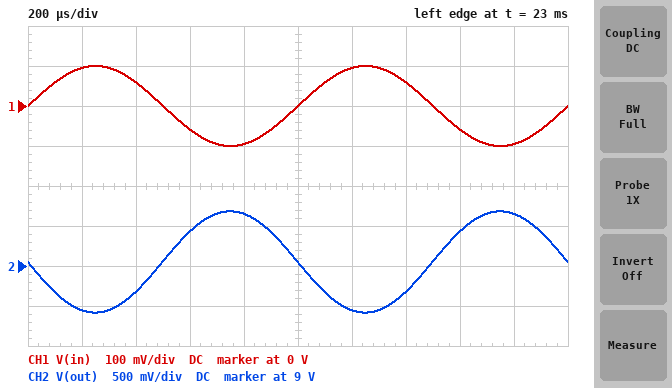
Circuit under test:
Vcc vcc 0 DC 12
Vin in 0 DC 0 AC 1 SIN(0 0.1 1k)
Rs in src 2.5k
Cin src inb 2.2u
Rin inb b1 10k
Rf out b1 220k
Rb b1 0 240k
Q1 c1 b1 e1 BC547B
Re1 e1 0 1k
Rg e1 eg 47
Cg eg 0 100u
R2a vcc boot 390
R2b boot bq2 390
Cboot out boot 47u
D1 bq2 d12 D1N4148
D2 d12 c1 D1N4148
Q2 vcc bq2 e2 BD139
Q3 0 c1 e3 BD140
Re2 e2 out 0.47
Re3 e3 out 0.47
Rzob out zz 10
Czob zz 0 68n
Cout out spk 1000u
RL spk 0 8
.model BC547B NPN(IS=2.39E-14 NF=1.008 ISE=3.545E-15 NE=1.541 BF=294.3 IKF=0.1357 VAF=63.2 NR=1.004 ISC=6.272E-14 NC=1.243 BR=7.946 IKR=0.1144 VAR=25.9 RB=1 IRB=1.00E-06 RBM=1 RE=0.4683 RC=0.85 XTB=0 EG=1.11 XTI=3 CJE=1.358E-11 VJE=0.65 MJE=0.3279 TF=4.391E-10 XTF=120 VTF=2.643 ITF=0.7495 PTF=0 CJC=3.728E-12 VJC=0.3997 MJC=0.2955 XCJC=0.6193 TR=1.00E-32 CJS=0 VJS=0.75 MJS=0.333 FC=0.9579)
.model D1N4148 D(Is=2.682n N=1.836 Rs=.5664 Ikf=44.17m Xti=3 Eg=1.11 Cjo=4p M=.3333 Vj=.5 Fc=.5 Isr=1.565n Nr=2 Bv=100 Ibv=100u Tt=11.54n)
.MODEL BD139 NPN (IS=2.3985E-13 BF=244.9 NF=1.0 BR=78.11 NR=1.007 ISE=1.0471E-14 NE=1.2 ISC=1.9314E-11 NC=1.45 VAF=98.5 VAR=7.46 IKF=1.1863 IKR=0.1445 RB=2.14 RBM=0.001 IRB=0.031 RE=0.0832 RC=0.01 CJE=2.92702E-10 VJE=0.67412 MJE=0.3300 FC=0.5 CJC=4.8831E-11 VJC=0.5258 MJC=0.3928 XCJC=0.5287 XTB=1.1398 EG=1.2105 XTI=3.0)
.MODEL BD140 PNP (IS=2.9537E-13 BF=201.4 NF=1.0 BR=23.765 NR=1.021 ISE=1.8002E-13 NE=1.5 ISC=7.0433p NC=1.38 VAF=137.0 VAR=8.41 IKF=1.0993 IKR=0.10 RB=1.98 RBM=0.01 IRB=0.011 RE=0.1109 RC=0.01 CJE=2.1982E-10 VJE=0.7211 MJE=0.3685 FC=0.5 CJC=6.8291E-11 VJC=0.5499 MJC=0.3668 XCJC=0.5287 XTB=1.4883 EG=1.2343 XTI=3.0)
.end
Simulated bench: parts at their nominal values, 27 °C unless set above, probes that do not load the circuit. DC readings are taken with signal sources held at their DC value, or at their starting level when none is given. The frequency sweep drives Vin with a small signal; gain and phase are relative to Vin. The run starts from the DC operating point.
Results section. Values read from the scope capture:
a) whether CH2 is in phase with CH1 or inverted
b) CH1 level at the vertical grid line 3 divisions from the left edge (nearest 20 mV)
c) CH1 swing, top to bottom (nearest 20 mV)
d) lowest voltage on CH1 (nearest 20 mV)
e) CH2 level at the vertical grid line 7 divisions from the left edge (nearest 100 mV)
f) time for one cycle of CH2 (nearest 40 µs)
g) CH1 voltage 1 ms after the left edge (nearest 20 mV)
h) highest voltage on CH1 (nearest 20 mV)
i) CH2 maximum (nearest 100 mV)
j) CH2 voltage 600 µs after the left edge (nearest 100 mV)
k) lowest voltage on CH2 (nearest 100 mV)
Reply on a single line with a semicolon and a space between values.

inverted; -60 mV; 200 mV; -100 mV; 8.7 V; 1.00 ms; 0 V; 100 mV; 9.7 V; 9.4 V; 8.4 V
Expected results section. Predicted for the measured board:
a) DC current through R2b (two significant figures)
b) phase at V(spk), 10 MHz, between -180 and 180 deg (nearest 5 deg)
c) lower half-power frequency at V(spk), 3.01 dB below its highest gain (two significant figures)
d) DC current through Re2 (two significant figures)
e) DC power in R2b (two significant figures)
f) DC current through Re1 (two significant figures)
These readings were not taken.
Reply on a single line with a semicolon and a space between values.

2.9 mA; 25 deg; 26 Hz; 23 mA; 3.3 mW; 2.9 mA
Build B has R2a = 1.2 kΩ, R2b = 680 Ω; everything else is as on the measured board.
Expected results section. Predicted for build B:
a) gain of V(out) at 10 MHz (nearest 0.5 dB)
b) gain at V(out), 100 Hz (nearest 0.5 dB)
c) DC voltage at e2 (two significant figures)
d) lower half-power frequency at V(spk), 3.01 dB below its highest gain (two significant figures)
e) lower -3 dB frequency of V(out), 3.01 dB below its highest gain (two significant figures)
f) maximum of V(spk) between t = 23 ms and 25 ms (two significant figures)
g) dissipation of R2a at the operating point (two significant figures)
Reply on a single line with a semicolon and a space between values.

-22.5 dB; 16.5 dB; 7.2 V; 17 Hz; 6.4 Hz; 670 mV; 5.9 mW
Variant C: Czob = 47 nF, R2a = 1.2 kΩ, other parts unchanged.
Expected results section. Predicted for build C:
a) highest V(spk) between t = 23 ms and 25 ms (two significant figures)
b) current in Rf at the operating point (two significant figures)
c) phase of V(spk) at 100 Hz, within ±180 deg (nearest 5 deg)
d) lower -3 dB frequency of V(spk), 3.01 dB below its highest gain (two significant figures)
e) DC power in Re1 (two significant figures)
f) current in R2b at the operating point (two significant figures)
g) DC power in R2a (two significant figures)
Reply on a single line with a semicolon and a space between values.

620 mV; 21 µA; -165 deg; 17 Hz; 5.7 mW; 2.4 mA; 6.7 mW
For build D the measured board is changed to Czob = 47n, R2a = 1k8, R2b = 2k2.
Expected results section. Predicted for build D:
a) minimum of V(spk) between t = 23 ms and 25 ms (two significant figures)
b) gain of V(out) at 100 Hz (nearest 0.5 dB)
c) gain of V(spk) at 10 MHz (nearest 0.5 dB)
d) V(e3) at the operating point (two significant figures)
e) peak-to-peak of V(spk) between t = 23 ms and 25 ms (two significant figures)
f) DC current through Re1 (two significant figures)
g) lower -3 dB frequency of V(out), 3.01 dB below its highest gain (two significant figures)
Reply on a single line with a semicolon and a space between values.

-690 mV; 17.0 dB; -28.0 dB; 5.3 V; 1.4 V; 1.5 mA; 3.7 Hz
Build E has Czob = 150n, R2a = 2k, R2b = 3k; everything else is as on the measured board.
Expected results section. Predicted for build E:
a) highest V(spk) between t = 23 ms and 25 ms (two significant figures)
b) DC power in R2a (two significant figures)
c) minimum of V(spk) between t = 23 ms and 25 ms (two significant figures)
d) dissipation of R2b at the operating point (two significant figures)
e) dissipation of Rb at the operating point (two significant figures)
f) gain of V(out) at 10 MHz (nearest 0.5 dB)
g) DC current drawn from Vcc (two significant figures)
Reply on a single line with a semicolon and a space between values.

700 mV; 3.5 mW; -680 mV; 5.2 mW; 16 µW; -30.5 dB; 8.0 mA
